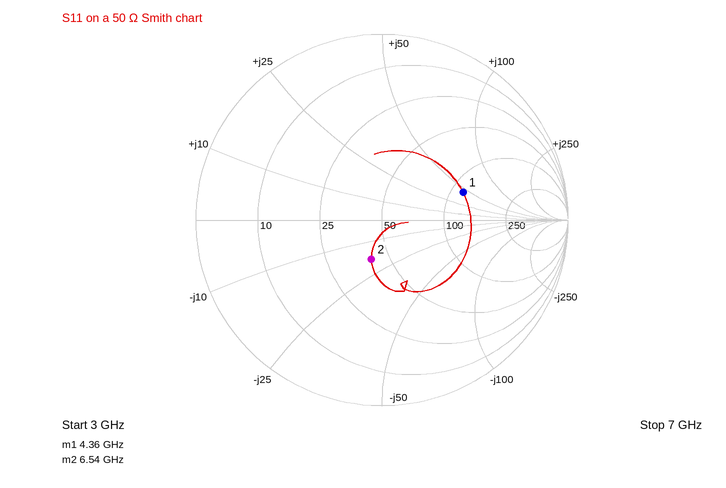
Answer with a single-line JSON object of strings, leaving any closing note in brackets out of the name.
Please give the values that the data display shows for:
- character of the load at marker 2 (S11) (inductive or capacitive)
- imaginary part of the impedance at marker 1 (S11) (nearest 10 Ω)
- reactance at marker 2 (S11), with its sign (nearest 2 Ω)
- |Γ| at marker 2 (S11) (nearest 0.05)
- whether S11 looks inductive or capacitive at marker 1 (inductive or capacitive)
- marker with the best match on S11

{"character of the load at marker 2 (S11)": "capacitive", "imaginary part of the impedance at marker 1 (S11)": "+40 Ω", "reactance at marker 2 (S11), with its sign": "-18 Ω", "|Γ| at marker 2 (S11)": "0.20", "whether S11 looks inductive or capacitive at marker 1": "inductive", "marker with the best match on S11": "marker 2"}
